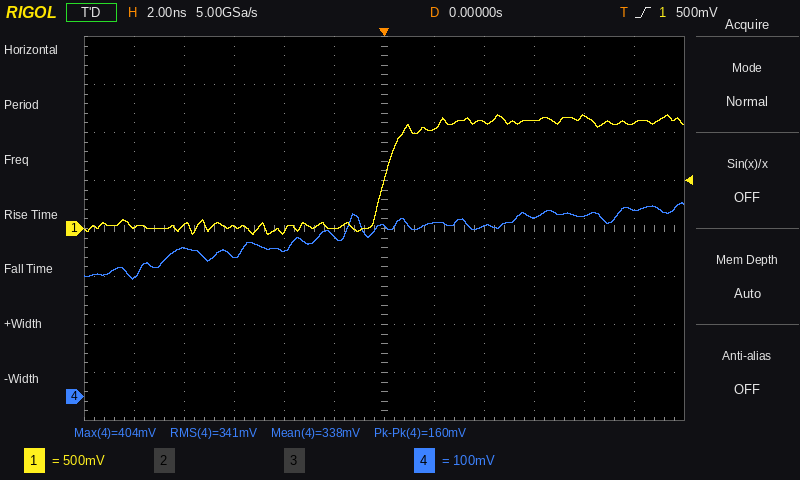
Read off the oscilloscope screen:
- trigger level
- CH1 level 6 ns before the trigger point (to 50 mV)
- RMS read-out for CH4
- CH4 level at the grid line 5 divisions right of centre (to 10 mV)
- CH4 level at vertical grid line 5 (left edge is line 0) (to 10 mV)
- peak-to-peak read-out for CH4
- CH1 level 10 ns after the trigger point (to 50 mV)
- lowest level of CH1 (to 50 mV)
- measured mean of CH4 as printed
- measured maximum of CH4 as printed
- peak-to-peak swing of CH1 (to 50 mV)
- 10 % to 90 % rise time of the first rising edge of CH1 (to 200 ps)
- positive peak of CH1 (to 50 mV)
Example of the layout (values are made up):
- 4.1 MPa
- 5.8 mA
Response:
- 500 mV
- 0 mV
- 341 mV
- 390 mV
- 330 mV
- 160 mV
- 1.10 V
- -50 mV
- 338 mV
- 404 mV
- 1.25 V
- 1.2 ns
- 1.20 V
